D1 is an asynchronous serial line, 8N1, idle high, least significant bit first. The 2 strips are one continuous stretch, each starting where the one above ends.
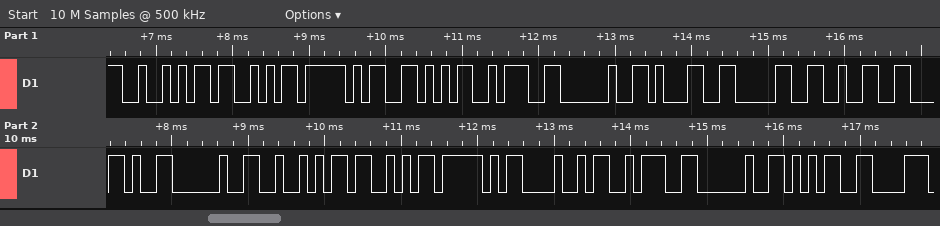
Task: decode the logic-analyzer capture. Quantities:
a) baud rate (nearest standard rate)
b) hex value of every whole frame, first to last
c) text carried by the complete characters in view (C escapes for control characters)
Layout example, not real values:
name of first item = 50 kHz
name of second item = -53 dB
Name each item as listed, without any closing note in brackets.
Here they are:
baud rate = 9600 baud
hex value of every whole frame, first to last = 52 53 5F 56 3A 20 31 30 32 2C 20 52 53 5F 48 3A 20 35
text carried by the complete characters in view = "RS_V: 102, RS_H: 5"
